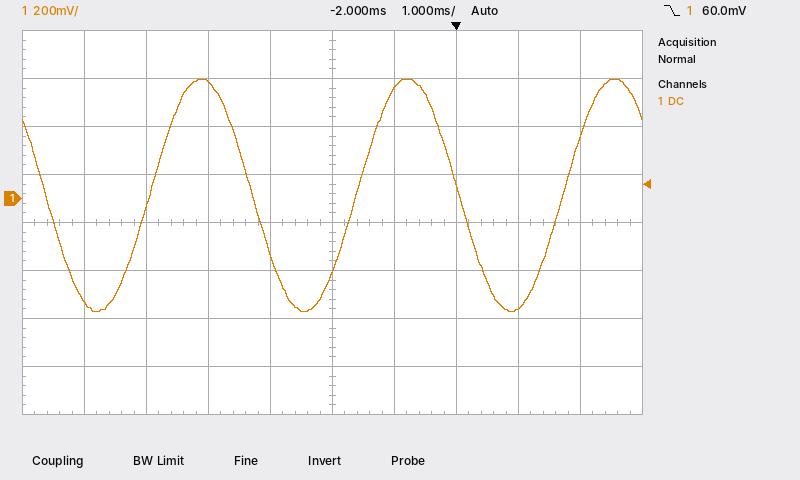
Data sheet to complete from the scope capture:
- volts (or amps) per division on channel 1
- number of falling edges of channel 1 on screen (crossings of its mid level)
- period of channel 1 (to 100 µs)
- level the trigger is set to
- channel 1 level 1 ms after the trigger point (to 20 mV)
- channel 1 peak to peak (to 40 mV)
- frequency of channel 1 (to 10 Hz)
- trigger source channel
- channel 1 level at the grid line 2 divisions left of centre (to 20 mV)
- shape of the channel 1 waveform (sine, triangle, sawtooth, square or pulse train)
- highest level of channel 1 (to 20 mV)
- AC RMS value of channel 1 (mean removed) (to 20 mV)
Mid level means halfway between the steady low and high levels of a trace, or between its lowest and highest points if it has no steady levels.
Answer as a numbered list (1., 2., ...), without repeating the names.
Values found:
1. 200 mV
2. 3
3. 3.3 ms
4. 60.0 mV
5. -460 mV
6. 960 mV
7. 300 Hz
8. channel 1
9. 480 mV
10. sine
11. 500 mV
12. 340 mV
